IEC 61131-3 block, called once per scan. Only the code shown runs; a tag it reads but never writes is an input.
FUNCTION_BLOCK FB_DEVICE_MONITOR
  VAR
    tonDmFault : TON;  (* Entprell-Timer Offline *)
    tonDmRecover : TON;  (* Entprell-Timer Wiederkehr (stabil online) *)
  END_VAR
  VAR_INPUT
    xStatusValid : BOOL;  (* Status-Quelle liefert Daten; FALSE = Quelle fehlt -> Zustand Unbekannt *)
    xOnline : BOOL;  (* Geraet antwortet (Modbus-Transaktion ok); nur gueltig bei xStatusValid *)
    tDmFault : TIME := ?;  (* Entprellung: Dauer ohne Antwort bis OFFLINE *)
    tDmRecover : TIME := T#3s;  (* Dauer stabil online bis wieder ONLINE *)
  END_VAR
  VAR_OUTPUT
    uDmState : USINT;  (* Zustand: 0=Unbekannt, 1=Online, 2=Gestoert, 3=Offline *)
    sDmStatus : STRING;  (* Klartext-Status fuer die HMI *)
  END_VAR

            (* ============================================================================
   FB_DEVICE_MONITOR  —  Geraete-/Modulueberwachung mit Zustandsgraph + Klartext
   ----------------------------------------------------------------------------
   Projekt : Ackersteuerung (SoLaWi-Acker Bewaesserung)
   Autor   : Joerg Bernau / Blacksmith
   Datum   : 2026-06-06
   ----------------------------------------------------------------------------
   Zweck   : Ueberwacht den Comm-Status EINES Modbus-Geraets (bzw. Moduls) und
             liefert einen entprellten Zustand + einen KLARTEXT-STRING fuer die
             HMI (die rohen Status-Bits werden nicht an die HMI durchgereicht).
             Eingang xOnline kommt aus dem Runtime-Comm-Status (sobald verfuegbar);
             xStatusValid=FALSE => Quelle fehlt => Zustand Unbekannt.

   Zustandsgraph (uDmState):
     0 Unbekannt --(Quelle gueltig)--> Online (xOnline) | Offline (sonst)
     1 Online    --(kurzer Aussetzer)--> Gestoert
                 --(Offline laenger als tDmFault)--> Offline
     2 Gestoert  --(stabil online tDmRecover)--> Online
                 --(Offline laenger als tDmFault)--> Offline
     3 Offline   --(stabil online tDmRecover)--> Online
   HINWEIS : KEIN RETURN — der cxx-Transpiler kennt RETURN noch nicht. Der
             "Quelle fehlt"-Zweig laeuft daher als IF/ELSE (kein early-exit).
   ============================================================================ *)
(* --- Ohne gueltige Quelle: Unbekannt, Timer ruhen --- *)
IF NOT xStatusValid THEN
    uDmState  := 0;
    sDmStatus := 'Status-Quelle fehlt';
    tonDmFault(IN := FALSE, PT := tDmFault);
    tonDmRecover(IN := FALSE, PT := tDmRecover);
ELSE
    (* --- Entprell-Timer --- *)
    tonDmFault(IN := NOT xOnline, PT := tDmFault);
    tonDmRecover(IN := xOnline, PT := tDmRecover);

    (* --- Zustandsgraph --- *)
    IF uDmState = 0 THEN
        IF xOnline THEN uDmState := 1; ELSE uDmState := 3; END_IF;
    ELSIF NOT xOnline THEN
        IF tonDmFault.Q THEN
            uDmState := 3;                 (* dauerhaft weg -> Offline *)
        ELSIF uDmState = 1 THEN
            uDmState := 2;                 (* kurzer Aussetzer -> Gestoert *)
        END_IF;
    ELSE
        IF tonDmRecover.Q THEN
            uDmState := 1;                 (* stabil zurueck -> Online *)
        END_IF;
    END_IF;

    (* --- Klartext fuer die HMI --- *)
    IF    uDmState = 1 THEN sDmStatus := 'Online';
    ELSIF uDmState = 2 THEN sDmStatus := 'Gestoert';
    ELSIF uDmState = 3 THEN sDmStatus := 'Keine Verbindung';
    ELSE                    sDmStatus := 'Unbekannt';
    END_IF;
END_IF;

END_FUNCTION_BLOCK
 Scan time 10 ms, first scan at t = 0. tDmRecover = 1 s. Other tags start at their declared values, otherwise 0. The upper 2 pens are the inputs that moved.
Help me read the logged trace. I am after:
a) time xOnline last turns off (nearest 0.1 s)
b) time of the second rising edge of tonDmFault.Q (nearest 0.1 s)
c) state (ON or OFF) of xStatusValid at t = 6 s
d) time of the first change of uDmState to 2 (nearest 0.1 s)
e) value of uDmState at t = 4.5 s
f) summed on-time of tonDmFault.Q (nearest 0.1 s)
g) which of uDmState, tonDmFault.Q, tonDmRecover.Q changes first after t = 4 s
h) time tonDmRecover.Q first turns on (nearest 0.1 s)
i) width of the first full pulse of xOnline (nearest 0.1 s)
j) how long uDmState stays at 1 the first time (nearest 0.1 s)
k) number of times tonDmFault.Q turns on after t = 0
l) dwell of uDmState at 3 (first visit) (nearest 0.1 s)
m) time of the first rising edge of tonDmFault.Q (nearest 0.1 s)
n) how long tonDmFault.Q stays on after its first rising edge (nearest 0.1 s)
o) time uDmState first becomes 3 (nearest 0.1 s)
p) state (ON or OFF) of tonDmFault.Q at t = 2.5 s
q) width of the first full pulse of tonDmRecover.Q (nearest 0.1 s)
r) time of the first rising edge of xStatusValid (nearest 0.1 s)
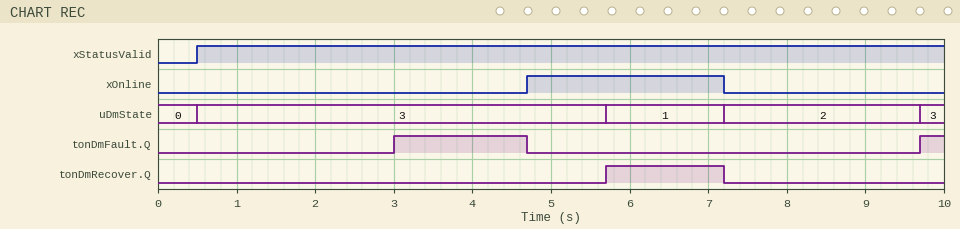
7.2 s
9.7 s
ON
7.2 s
3
2.0 s
tonDmFault.Q
5.7 s
2.5 s
1.5 s
2
5.2 s
3.0 s
1.7 s
0.5 s
OFF
1.5 s
0.5 s
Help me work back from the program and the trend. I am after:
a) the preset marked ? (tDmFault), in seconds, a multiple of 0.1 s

2.5 s
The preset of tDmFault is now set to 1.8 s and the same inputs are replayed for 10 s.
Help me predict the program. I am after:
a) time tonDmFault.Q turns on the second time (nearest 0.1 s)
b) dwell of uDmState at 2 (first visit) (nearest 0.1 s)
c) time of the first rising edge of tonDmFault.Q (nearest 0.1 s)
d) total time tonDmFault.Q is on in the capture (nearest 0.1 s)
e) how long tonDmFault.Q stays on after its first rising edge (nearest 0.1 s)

9.0 s
1.8 s
2.3 s
3.4 s
2.4 s
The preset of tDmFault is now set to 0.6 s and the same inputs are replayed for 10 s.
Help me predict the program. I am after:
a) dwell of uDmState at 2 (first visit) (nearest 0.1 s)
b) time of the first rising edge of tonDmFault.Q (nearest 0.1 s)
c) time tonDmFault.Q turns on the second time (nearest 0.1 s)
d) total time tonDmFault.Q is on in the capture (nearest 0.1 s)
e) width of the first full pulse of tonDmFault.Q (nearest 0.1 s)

0.6 s
1.1 s
7.8 s
5.8 s
3.6 s
